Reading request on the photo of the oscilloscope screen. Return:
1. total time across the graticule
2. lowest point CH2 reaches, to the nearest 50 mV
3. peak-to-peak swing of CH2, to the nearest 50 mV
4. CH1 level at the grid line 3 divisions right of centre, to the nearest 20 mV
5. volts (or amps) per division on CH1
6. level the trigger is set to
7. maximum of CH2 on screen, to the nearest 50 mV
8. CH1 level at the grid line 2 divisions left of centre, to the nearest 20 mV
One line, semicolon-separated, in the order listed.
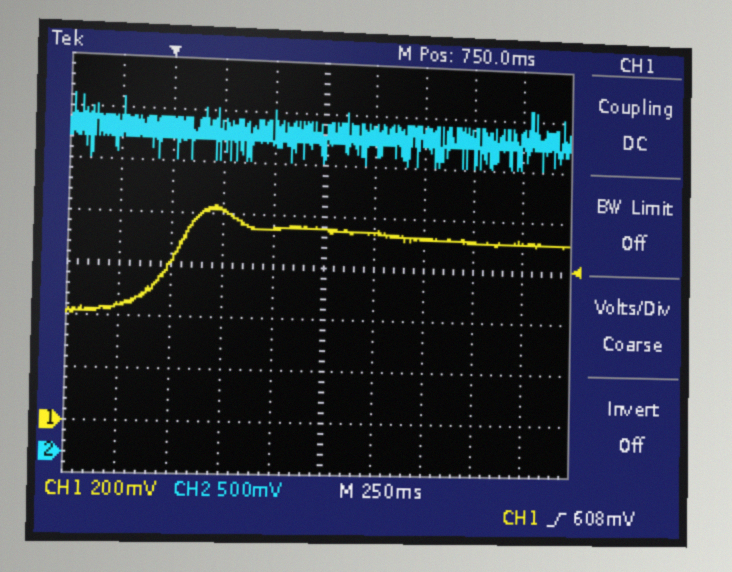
2.5 s; 2.80 V; 600 mV; 720 mV; 200 mV; 608 mV; 3.40 V; 820 mV
